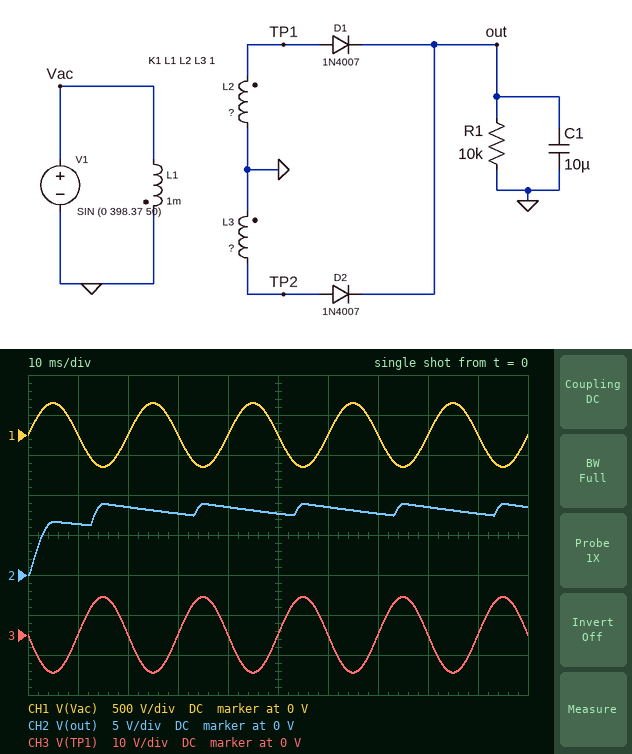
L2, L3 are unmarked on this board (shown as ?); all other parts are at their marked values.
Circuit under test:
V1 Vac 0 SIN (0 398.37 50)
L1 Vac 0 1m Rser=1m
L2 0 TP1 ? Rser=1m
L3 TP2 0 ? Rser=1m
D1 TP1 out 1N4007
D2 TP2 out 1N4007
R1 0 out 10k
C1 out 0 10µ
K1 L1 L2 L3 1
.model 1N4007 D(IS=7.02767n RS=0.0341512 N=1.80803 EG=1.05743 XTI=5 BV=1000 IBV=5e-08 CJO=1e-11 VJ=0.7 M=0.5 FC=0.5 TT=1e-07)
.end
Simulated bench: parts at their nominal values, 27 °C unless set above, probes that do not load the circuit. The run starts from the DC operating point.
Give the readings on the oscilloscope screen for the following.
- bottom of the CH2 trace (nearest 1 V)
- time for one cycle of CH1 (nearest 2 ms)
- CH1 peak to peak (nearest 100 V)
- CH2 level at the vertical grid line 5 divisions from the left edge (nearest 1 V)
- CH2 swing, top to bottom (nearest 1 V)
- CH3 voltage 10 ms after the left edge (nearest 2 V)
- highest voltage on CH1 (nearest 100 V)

0 V
20 ms
800 V
8 V
9 V
0 V
400 V
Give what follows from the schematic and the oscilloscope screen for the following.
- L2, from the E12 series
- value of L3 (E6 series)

560 nH
330 nH
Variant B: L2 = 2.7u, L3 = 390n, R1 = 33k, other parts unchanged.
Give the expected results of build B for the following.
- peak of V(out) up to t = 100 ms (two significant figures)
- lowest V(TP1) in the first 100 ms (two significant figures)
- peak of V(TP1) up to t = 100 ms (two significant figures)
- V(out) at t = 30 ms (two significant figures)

20 V
-21 V
21 V
19 V
